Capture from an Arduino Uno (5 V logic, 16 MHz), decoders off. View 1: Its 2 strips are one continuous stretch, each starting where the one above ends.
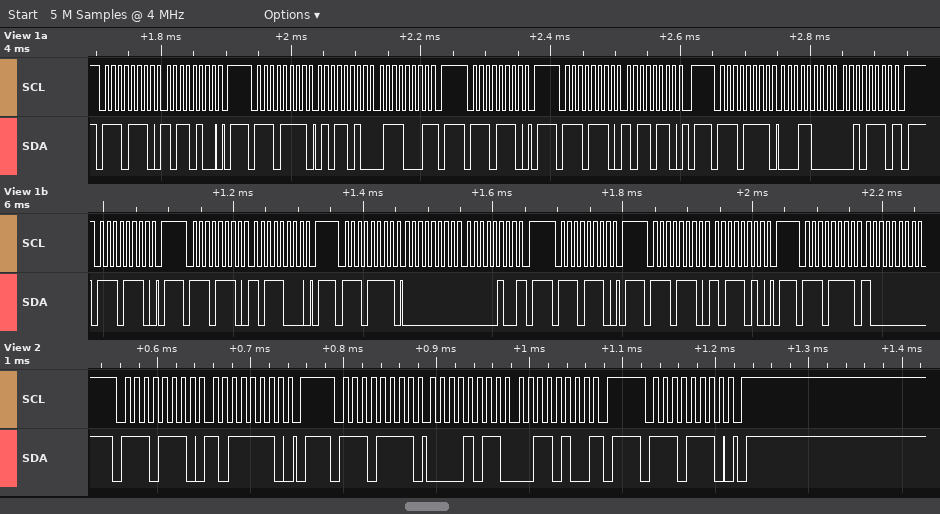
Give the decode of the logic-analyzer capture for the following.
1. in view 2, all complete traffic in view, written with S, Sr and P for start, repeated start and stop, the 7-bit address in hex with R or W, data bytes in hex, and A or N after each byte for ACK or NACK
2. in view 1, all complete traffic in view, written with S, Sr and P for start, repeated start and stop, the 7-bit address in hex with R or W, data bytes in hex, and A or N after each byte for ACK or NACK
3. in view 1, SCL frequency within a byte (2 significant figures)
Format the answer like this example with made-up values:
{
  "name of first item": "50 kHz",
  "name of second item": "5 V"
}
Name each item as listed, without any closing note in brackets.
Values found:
{
  "in view 2, all complete traffic in view, written with S, Sr and P for start, repeated start and stop, the 7-bit address in hex with R or W, data bytes in hex, and A or N after each byte for ACK or NACK": "S 77W A BE A P S 77R A 0B A 34 N P S 77W A P",
  "in view 1, all complete traffic in view, written with S, Sr and P for start, repeated start and stop, the 7-bit address in hex with R or W, data bytes in hex, and A or N after each byte for ACK or NACK": "S 77W A B4 A P S 77R A 5A A 71 N P S 77W A P S 77W A B6 A P S 77R A 18 A 2E N P S 77W A P S 77W A B8 A P S 77R A 00 A 04 N P S 77W A P S 77W A BA A P S 77R A 80 A",
  "in view 1, SCL frequency within a byte": "100 kHz"
}
